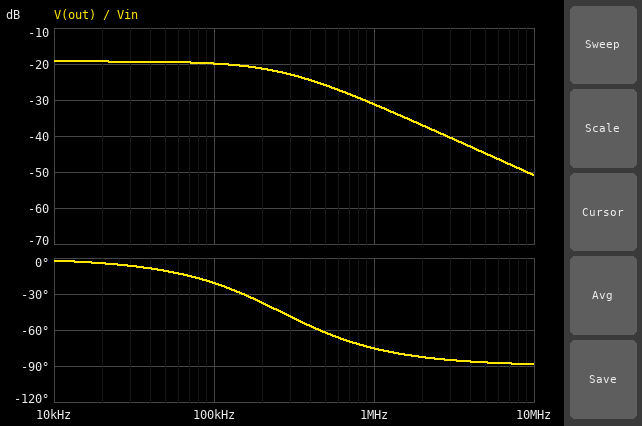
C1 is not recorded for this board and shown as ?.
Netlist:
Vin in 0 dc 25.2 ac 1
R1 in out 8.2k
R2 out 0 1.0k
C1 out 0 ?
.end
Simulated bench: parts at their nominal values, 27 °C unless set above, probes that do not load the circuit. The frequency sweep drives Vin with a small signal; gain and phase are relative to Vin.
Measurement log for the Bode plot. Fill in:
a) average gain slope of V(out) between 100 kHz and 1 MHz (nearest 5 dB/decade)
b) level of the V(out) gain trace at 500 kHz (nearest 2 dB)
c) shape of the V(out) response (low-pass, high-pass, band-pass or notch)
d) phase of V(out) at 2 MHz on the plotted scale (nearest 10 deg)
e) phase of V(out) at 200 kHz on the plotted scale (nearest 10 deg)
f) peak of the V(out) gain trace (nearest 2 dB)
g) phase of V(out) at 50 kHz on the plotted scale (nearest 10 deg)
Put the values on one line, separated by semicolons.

-10 dB/decade; -26 dB; low-pass; -80 deg; -40 deg; -20 dB; -10 deg
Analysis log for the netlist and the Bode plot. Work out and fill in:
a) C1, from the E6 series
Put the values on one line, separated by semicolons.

680 pF
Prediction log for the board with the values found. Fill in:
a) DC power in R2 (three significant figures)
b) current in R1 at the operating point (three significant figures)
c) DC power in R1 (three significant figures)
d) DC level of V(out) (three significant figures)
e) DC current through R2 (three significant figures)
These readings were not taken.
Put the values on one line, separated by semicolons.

7.50 mW; 2.74 mA; 61.5 mW; 2.74 V; 2.74 mA
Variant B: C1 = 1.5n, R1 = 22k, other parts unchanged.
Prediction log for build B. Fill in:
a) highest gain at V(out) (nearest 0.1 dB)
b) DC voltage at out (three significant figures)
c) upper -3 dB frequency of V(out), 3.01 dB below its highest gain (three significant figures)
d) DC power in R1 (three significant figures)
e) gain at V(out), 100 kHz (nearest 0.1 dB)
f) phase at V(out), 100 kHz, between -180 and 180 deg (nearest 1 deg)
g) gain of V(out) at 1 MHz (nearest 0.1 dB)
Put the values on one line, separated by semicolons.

-27.2 dB; 1.10 V; 111 kHz; 26.4 mW; -29.8 dB; -42 deg; -46.4 dB
